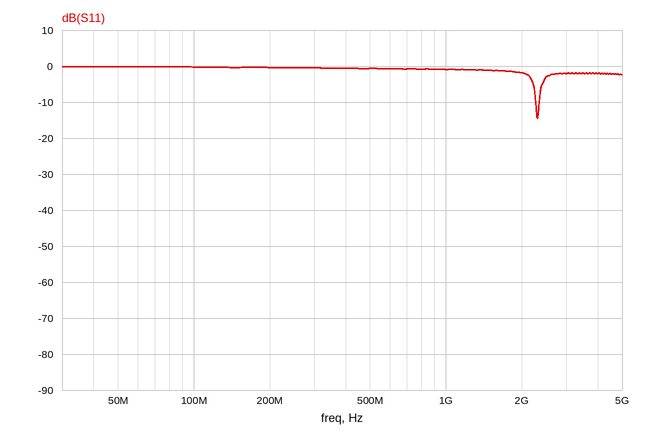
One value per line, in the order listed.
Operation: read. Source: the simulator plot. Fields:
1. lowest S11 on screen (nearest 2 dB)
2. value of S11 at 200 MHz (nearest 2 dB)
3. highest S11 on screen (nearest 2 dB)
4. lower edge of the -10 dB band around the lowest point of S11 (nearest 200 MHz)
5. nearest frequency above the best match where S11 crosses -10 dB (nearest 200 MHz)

-14 dB
0 dB
0 dB
2.2 GHz
2.4 GHz
